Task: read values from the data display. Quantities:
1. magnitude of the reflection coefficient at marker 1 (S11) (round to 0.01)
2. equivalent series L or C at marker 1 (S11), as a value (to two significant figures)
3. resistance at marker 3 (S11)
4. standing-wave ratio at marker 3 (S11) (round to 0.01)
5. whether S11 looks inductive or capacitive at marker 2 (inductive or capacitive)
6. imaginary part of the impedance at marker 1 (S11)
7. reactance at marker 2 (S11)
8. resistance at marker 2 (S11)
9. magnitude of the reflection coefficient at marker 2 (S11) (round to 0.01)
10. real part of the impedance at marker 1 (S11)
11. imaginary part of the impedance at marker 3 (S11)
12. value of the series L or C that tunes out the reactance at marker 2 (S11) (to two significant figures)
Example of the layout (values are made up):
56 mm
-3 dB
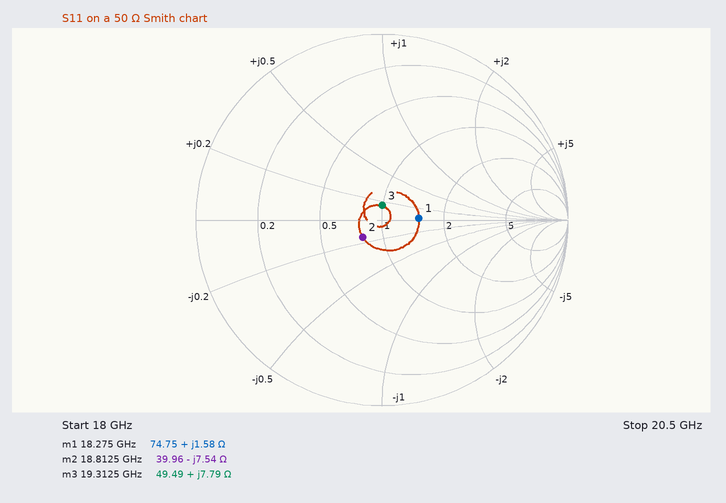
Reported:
0.20
14 pH
49.49 Ω
1.17
capacitive
+1.58 Ω
-7.54 Ω
39.96 Ω
0.14
74.75 Ω
+7.79 Ω
64 pH
